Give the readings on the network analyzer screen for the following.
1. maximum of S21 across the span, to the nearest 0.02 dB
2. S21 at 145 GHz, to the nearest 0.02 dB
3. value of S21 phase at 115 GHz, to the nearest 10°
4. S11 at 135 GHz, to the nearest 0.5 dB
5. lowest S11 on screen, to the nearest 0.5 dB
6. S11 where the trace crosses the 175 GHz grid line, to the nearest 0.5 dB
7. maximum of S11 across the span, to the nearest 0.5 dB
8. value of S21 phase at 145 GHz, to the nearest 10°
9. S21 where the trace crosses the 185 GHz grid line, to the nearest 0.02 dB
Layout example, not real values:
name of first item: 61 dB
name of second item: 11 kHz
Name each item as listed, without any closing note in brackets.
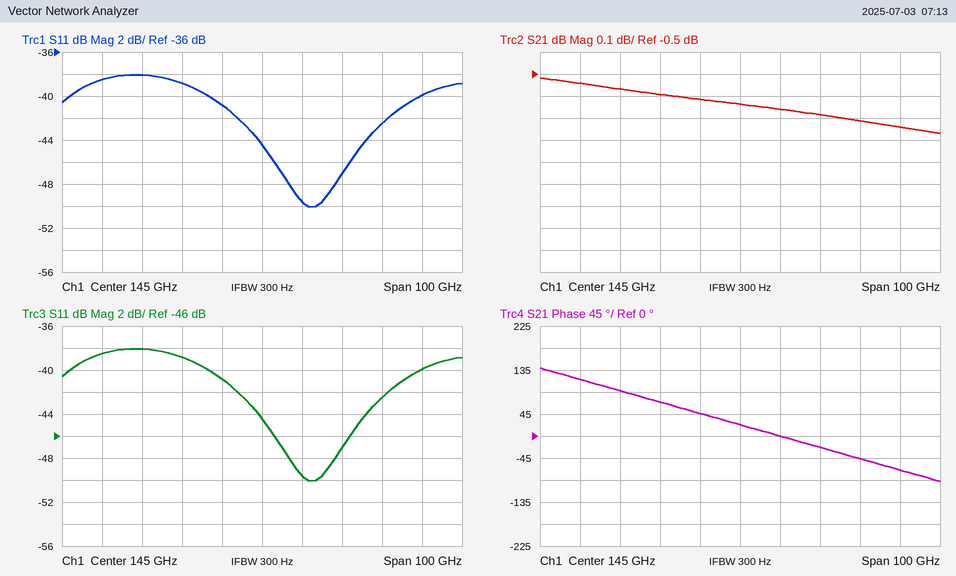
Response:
maximum of S21 across the span, to the nearest 0.02 dB: -0.52 dB
S21 at 145 GHz, to the nearest 0.02 dB: -0.64 dB
value of S21 phase at 115 GHz, to the nearest 10°: 90°
S11 at 135 GHz, to the nearest 0.5 dB: -41.0 dB
lowest S11 on screen, to the nearest 0.5 dB: -50.0 dB
S11 where the trace crosses the 175 GHz grid line, to the nearest 0.5 dB: -42.5 dB
maximum of S11 across the span, to the nearest 0.5 dB: -38.0 dB
value of S21 phase at 145 GHz, to the nearest 10°: 20°
S21 where the trace crosses the 185 GHz grid line, to the nearest 0.02 dB: -0.74 dB
